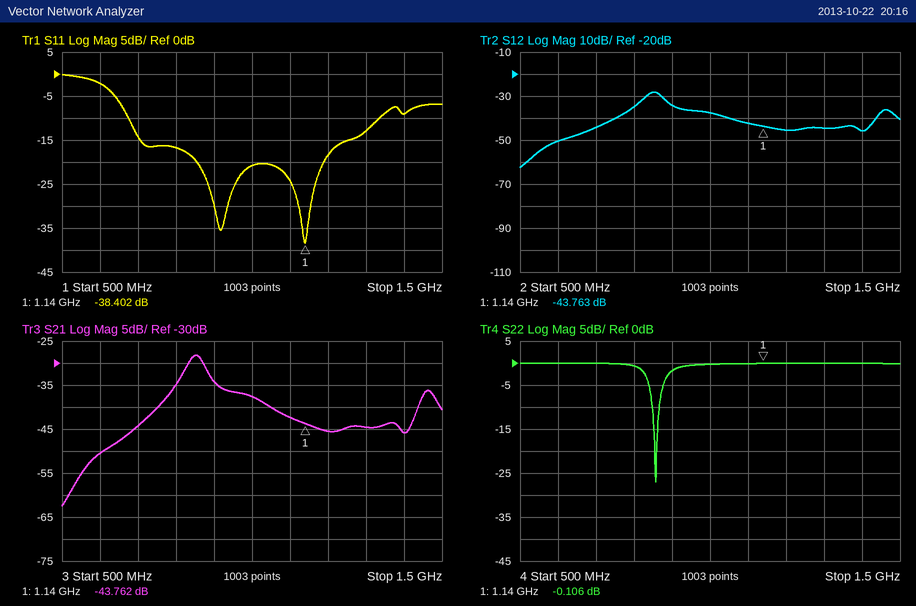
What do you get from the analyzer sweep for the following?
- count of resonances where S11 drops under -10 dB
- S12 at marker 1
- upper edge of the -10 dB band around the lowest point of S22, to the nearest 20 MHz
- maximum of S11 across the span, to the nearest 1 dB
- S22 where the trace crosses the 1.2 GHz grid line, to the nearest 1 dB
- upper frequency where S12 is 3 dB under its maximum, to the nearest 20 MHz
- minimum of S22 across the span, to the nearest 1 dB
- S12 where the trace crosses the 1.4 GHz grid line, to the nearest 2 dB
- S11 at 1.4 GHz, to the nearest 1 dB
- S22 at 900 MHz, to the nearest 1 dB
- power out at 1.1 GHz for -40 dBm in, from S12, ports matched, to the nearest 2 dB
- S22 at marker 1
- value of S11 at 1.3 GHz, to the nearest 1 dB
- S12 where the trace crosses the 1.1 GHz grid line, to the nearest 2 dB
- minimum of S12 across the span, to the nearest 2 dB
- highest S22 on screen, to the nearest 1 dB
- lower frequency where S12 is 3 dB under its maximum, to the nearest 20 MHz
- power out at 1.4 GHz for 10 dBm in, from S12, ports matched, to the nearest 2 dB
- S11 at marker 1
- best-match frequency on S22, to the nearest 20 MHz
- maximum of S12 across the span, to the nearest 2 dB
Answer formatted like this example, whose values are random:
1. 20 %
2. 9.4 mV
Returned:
1. 2
2. -43.763 dB
3. 860 MHz
4. 0 dB
5. 0 dB
6. 880 MHz
7. -27 dB
8. -46 dB
9. -9 dB
10. -2 dB
11. -82 dBm
12. -0.106 dB
13. -13 dB
14. -42 dB
15. -62 dB
16. 0 dB
17. 820 MHz
18. -36 dBm
19. -38.402 dB
20. 860 MHz
21. -28 dB
